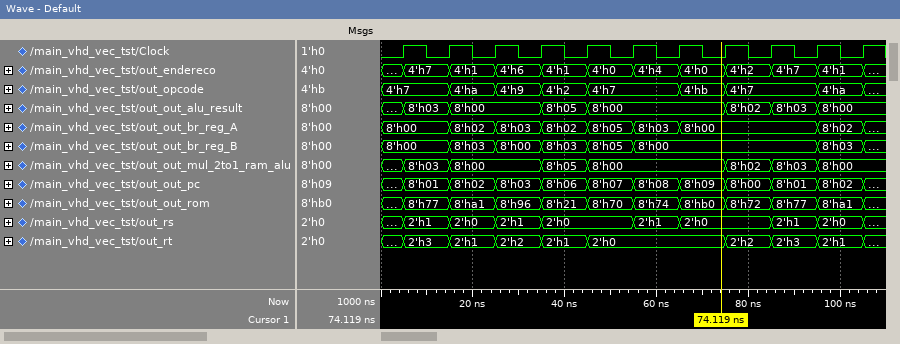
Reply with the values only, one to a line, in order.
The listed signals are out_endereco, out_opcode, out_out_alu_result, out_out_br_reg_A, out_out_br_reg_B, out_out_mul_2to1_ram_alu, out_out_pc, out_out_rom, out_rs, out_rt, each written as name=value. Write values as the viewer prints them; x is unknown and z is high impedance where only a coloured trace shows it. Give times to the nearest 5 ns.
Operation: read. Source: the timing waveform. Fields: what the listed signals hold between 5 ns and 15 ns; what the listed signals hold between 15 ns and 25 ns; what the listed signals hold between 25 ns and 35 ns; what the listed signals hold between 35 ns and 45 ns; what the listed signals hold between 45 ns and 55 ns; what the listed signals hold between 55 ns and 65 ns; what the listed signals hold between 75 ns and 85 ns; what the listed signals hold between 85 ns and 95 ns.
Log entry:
out_endereco=4'h7, out_opcode=4'h7, out_out_alu_result=8'h03, out_out_br_reg_A=8'h00, out_out_br_reg_B=8'h00, out_out_mul_2to1_ram_alu=8'h03, out_out_pc=8'h01, out_out_rom=8'h77, out_rs=2'h1, out_rt=2'h3
out_endereco=4'h1, out_opcode=4'ha, out_out_alu_result=8'h00, out_out_br_reg_A=8'h02, out_out_br_reg_B=8'h03, out_out_mul_2to1_ram_alu=8'h00, out_out_pc=8'h02, out_out_rom=8'ha1, out_rs=2'h0, out_rt=2'h1
out_endereco=4'h6, out_opcode=4'h9, out_out_alu_result=8'h00, out_out_br_reg_A=8'h03, out_out_br_reg_B=8'h00, out_out_mul_2to1_ram_alu=8'h00, out_out_pc=8'h03, out_out_rom=8'h96, out_rs=2'h1, out_rt=2'h2
out_endereco=4'h1, out_opcode=4'h2, out_out_alu_result=8'h05, out_out_br_reg_A=8'h02, out_out_br_reg_B=8'h03, out_out_mul_2to1_ram_alu=8'h05, out_out_pc=8'h06, out_out_rom=8'h21, out_rs=2'h0, out_rt=2'h1
out_endereco=4'h0, out_opcode=4'h7, out_out_alu_result=8'h00, out_out_br_reg_A=8'h05, out_out_br_reg_B=8'h05, out_out_mul_2to1_ram_alu=8'h00, out_out_pc=8'h07, out_out_rom=8'h70, out_rs=2'h0, out_rt=2'h0
out_endereco=4'h4, out_opcode=4'h7, out_out_alu_result=8'h00, out_out_br_reg_A=8'h03, out_out_br_reg_B=8'h00, out_out_mul_2to1_ram_alu=8'h00, out_out_pc=8'h08, out_out_rom=8'h74, out_rs=2'h1, out_rt=2'h0
out_endereco=4'h2, out_opcode=4'h7, out_out_alu_result=8'h02, out_out_br_reg_A=8'h00, out_out_br_reg_B=8'h00, out_out_mul_2to1_ram_alu=8'h02, out_out_pc=8'h00, out_out_rom=8'h72, out_rs=2'h0, out_rt=2'h2
out_endereco=4'h7, out_opcode=4'h7, out_out_alu_result=8'h03, out_out_br_reg_A=8'h00, out_out_br_reg_B=8'h00, out_out_mul_2to1_ram_alu=8'h03, out_out_pc=8'h01, out_out_rom=8'h77, out_rs=2'h1, out_rt=2'h3
